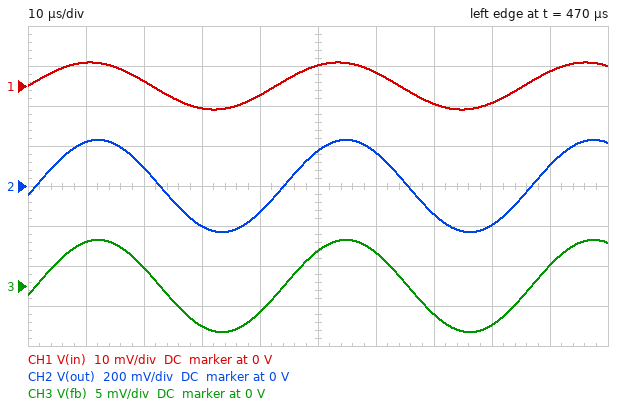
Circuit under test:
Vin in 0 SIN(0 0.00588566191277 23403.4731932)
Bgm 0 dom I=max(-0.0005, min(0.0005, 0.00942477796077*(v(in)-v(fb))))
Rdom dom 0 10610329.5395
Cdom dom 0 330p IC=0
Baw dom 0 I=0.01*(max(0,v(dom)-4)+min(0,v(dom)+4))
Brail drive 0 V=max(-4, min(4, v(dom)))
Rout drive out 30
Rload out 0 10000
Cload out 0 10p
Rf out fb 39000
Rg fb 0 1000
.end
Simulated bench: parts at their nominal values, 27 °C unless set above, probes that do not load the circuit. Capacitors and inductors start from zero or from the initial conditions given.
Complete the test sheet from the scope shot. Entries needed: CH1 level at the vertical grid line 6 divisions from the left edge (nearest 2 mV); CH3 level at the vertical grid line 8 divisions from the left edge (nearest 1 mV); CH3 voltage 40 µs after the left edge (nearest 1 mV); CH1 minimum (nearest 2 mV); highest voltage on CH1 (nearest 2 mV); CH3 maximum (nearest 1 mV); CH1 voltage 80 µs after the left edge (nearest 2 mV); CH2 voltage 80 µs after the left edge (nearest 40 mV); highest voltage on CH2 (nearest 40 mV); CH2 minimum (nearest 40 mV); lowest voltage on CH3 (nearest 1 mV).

4 mV
-5 mV
-3 mV
-6 mV
6 mV
6 mV
-4 mV
-200 mV
240 mV
-240 mV
-6 mV
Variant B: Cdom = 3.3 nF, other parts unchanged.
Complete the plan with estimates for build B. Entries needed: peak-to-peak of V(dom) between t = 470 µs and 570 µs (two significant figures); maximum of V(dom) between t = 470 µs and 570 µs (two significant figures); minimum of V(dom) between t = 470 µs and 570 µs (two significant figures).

210 mV
100 mV
-100 mV
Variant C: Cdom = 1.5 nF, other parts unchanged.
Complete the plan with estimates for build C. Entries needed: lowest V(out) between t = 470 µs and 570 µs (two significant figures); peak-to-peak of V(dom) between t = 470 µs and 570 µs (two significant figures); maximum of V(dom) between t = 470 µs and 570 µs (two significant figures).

-170 mV
340 mV
170 mV
